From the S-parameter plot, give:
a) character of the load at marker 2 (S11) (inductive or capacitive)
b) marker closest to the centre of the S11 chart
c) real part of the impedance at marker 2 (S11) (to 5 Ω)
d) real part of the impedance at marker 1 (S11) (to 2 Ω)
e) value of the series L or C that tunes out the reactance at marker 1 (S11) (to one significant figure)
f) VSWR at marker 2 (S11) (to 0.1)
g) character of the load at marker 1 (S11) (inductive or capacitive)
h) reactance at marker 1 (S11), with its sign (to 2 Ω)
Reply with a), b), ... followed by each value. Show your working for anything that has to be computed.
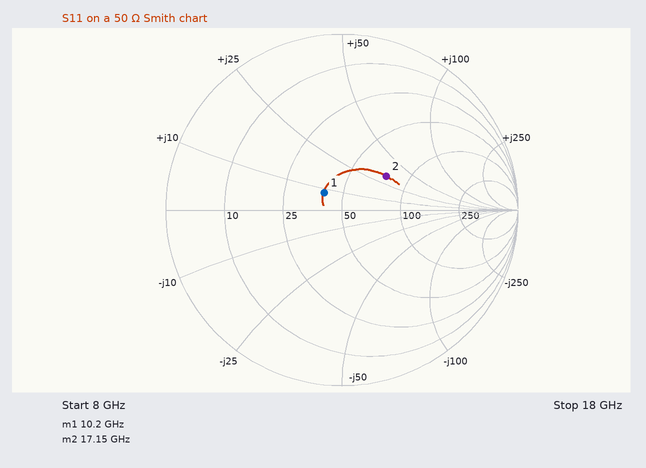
a) inductive
b) marker 1
c) 75 Ω
d) 40 Ω
e) C = 1/(2π × 10.2 GHz × 8 Ω) ≈ 2 pF
f) 1.9
g) inductive
h) +8 Ω
